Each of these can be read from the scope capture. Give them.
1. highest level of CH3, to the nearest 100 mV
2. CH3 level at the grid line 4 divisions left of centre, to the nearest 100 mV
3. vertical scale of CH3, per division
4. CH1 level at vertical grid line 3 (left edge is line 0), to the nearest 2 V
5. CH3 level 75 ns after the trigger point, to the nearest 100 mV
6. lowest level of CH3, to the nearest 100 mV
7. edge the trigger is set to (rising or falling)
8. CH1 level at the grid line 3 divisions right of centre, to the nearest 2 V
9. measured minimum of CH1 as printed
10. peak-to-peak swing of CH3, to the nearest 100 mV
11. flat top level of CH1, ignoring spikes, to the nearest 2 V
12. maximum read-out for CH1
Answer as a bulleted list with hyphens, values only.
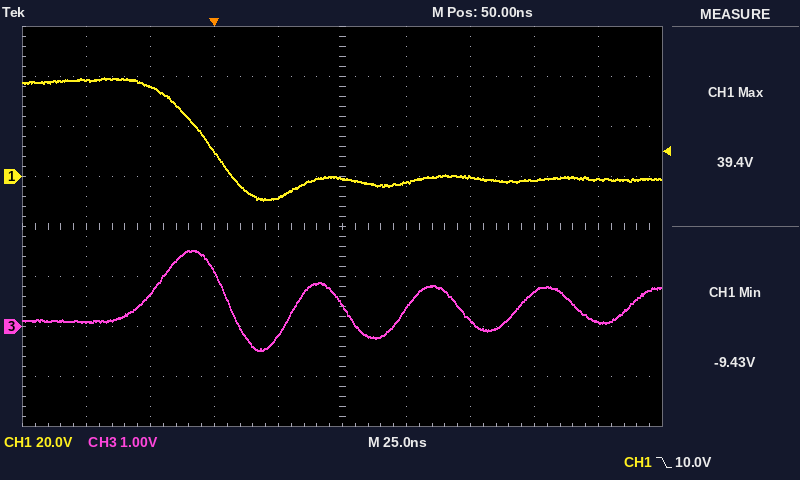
- 1.5 V
- 100 mV
- 1 V
- 10 V
- 400 mV
- -500 mV
- falling
- -2 V
- -9.43 V
- 2.0 V
- 38 V
- 39.4 V
